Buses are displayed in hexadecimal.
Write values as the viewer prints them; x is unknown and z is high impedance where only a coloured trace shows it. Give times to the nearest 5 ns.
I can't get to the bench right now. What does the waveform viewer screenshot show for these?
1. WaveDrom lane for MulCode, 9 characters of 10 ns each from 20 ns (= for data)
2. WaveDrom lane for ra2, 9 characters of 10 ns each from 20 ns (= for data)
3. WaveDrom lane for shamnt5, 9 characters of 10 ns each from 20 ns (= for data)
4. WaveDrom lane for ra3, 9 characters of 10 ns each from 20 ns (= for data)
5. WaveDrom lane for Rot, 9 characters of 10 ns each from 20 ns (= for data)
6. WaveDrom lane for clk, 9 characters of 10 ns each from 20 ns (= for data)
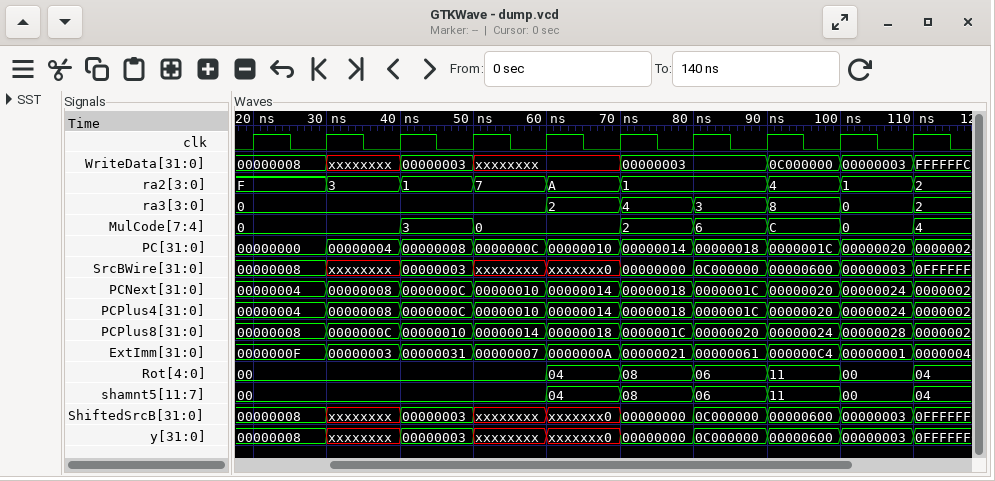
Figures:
{name: 'MulCode', wave: '=.==.====', data: '0 3 0 2 6 C 0'}
{name: 'ra2', wave: '======.==', data: 'F 3 1 7 A 1 4 1'}
{name: 'shamnt5', wave: '=...=====', data: '00 04 08 06 11 00'}
{name: 'ra3', wave: '=...=====', data: '0 2 4 3 8 0'}
{name: 'Rot', wave: '=...=====', data: '00 04 08 06 11 00'}
{name: 'clk', wave: 'p........'}
